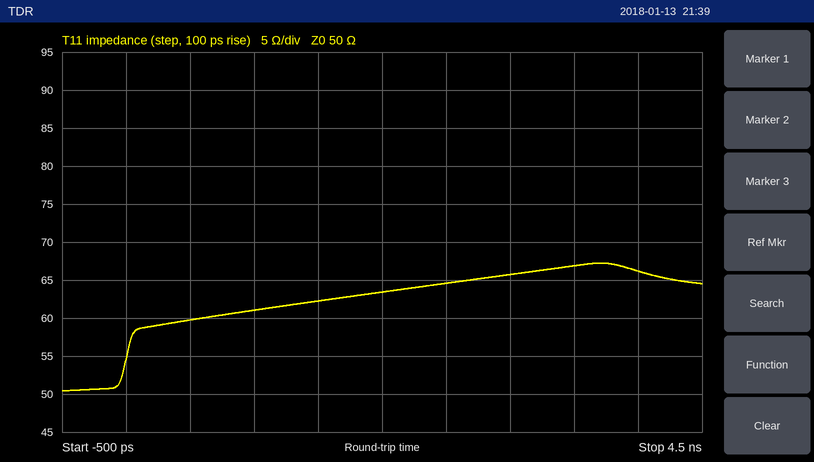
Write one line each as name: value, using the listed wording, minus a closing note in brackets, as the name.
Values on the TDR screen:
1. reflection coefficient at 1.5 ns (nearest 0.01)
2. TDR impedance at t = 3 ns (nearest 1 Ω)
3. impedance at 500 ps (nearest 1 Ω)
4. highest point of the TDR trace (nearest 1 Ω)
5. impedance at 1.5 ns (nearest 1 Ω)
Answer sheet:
reflection coefficient at 1.5 ns: +0.11
TDR impedance at t = 3 ns: 66 Ω
impedance at 500 ps: 60 Ω
highest point of the TDR trace: 67 Ω
impedance at 1.5 ns: 62 Ω
